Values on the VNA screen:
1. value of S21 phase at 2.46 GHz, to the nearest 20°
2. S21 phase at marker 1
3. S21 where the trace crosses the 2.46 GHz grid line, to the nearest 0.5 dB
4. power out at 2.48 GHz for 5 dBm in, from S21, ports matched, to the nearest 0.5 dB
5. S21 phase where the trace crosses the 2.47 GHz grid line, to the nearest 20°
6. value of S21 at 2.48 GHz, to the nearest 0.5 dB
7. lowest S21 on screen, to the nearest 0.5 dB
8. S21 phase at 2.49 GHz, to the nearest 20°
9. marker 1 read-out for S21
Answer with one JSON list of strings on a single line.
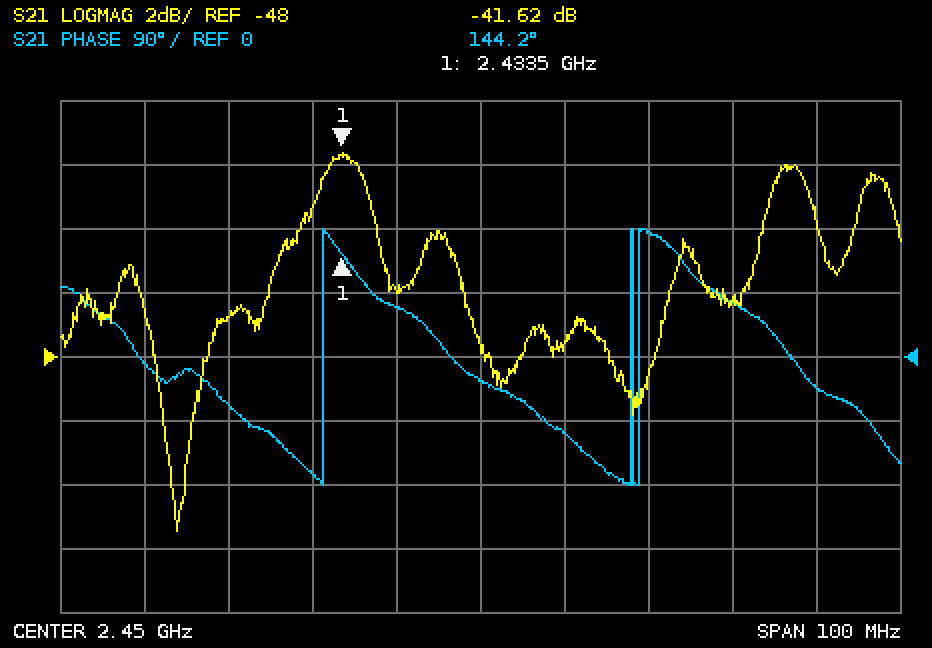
["-100°", "144.2°", "-47.5 dB", "-41.0 dBm", "180°", "-46.0 dB", "-53.5 dB", "-40°", "-41.62 dB"]
